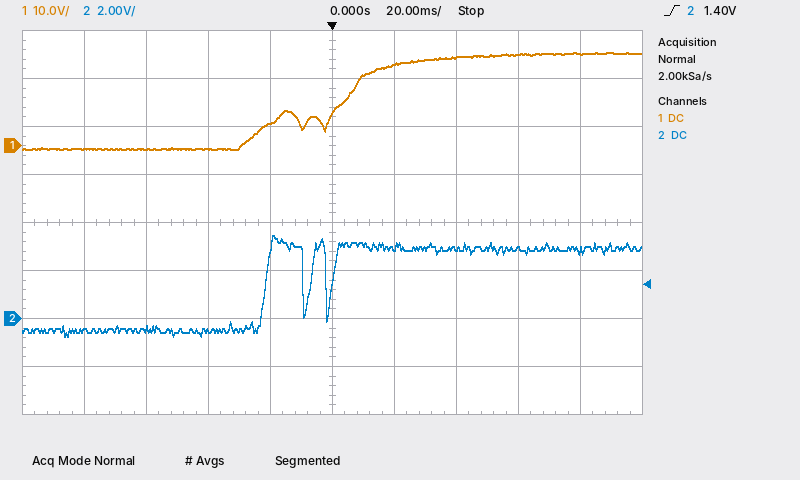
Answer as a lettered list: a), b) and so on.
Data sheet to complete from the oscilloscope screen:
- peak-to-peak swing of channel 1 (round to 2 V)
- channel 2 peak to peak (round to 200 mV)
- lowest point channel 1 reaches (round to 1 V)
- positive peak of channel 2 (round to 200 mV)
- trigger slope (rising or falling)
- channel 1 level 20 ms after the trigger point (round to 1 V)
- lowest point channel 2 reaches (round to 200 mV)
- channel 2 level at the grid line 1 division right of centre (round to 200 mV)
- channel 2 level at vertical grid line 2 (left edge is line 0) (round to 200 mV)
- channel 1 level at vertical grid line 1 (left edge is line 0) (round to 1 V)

a) 20 V
b) 4.2 V
c) -1 V
d) 3.4 V
e) rising
f) 17 V
g) -800 mV
h) 3.0 V
i) -400 mV
j) -1 V
